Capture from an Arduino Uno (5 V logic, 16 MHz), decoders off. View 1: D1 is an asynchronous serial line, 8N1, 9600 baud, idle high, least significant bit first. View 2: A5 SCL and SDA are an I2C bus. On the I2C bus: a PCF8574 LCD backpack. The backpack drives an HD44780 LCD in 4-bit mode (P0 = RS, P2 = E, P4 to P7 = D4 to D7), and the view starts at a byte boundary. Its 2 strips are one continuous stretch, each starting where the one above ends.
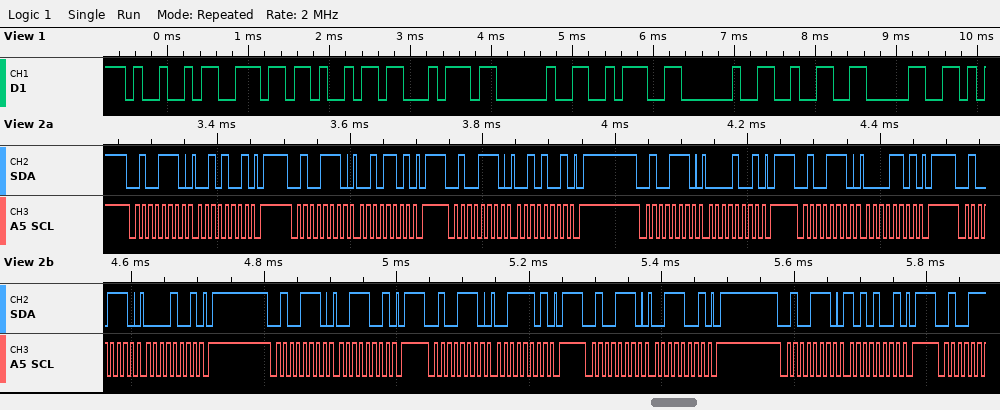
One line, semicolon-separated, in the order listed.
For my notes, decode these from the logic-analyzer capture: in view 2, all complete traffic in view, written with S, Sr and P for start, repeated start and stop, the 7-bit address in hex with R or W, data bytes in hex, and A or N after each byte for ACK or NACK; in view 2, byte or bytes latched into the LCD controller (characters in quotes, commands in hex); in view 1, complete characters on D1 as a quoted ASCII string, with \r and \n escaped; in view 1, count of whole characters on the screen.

S 27W A 29 A P S 27W A 2D A P S 27W A 29 A P S 27W A 09 A P S 27W A 0D A P S 27W A 09 A P S 27W A 39 A P S 27W A 3D A P S 27W A 39 A P S 27W A A9 A P; ' '; "Init : 20"; 9
